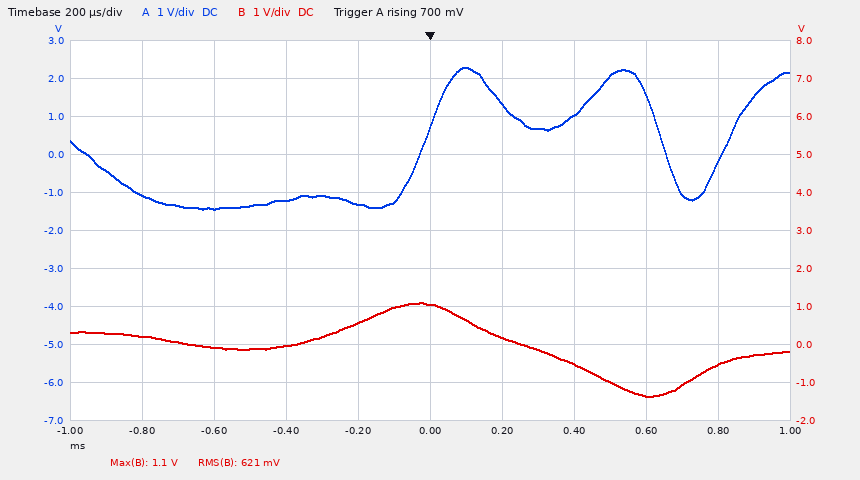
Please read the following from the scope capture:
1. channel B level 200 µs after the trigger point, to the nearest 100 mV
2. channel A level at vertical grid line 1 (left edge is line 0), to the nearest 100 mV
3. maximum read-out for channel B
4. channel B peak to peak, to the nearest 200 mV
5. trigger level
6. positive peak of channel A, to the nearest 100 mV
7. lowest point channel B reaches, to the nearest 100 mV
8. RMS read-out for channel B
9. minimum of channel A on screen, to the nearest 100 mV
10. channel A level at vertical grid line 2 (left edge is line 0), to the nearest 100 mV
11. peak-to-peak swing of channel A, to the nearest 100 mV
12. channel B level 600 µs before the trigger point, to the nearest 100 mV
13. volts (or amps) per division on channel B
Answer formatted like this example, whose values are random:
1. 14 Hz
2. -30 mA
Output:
1. 200 mV
2. -1.1 V
3. 1.1 V
4. 2.4 V
5. 700 mV
6. 2.3 V
7. -1.4 V
8. 621 mV
9. -1.4 V
10. -1.4 V
11. 3.7 V
12. -100 mV
13. 1 V
